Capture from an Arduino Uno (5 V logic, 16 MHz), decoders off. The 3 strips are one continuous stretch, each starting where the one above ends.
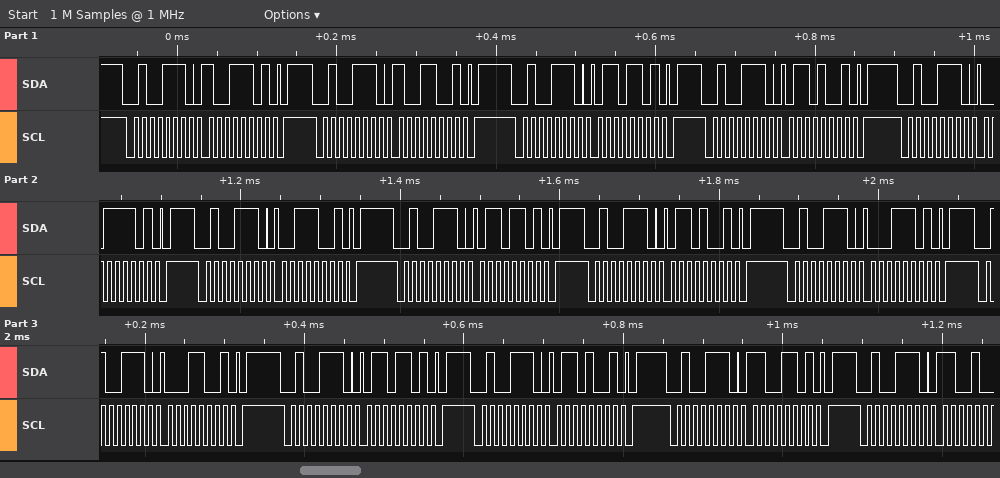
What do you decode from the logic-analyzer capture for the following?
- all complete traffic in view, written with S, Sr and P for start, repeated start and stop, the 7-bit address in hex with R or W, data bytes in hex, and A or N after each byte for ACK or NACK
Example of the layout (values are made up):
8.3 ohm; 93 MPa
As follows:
S 27W A 9D A P S 27W A 99 A P S 27W A 6D A P S 27W A 69 A P S 27W A 3D A P S 27W A 39 A P S 27W A 6D A P S 27W A 69 A P S 27W A 1D A P S 27W A 19 A P S 27W A 6D A P S 27W A 69 A P S 27W A CD A P S 27W A
